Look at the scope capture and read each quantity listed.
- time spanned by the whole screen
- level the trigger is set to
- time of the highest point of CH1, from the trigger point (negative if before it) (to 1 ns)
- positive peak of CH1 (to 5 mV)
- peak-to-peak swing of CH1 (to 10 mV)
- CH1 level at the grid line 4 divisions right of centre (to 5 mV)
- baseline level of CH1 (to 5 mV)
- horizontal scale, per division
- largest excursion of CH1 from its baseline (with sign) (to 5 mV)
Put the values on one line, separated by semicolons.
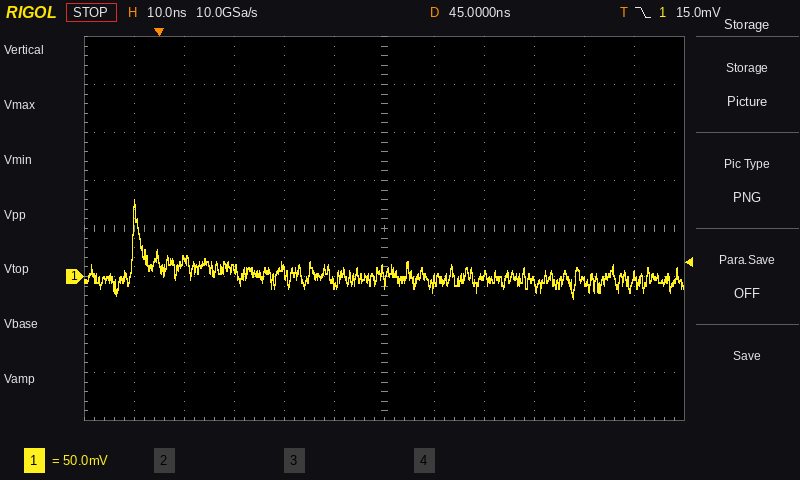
120 ns; 15.0 mV; -5 ns; 80 mV; 100 mV; -5 mV; 0 mV; 10 ns; +80 mV
